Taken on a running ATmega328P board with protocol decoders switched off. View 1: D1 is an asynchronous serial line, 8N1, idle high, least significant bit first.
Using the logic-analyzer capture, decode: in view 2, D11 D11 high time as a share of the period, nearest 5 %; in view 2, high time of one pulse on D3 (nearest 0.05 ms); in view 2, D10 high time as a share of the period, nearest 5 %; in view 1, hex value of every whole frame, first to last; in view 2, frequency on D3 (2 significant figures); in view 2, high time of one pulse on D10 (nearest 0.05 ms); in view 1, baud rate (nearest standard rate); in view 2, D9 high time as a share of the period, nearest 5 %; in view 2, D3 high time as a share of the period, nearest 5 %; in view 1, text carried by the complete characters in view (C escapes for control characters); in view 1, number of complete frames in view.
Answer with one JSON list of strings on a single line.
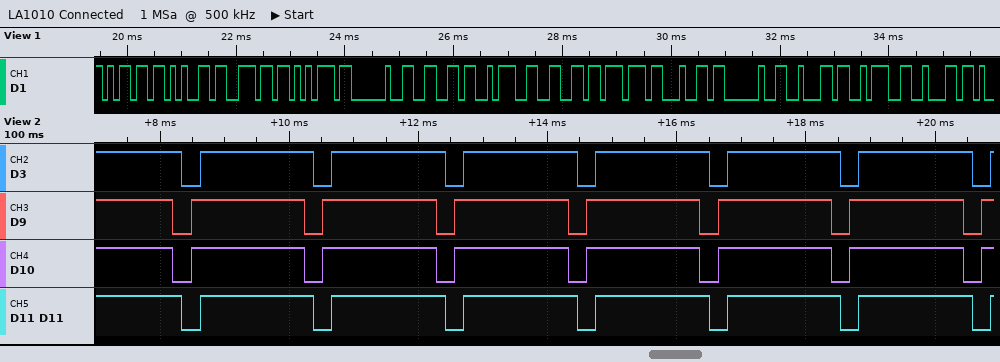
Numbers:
["85 %", "1.75 ms", "85 %", "0x6D 0x65 0x6E 0x75 0x20 0x66 0x3A 0x66 0x77 0x64 0x20 0x62 0x3A 0x62", "490 Hz", "1.75 ms", "9600 baud", "85 %", "85 %", "\"menu f:fwd b:b\"", "14"]
